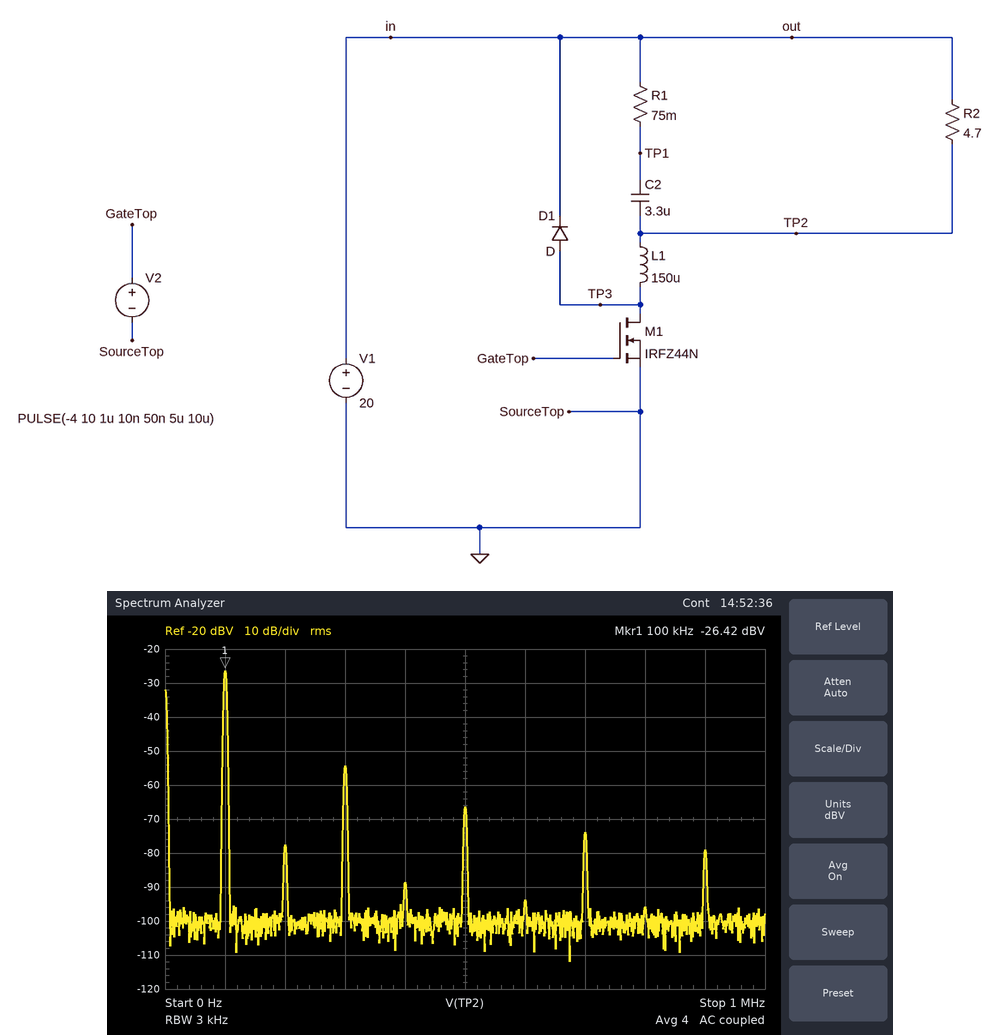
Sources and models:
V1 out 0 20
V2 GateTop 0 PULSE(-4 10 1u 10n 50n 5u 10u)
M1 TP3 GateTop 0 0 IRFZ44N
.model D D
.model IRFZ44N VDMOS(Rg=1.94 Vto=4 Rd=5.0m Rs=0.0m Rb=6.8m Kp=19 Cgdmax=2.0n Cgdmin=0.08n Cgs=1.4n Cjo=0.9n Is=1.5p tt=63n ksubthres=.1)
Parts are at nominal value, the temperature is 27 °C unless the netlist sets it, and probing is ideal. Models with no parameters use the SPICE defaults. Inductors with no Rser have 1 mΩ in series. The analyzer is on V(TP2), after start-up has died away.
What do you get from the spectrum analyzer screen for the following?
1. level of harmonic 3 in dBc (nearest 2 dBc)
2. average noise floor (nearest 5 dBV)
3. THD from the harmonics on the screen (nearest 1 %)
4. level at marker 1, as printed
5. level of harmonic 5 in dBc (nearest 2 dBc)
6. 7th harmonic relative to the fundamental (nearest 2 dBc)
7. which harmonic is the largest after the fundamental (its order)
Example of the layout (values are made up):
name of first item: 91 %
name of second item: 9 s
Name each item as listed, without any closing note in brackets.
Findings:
level of harmonic 3 in dBc: -28 dBc
average noise floor: -100 dBV
THD from the harmonics on the screen: 4 %
level at marker 1, as printed: -26.42 dBV
level of harmonic 5 in dBc: -40 dBc
7th harmonic relative to the fundamental: -48 dBc
which harmonic is the largest after the fundamental: 3
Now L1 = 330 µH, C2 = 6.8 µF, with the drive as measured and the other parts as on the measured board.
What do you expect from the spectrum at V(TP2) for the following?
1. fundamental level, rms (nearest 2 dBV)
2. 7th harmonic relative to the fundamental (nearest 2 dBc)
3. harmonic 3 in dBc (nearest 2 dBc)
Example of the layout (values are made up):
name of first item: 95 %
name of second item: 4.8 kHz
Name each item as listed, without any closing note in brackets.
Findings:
fundamental level, rms: -40 dBV
7th harmonic relative to the fundamental: -44 dBc
harmonic 3 in dBc: -26 dBc
